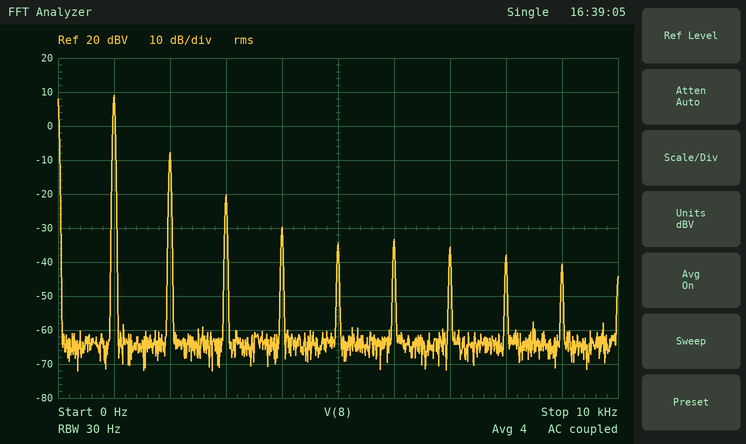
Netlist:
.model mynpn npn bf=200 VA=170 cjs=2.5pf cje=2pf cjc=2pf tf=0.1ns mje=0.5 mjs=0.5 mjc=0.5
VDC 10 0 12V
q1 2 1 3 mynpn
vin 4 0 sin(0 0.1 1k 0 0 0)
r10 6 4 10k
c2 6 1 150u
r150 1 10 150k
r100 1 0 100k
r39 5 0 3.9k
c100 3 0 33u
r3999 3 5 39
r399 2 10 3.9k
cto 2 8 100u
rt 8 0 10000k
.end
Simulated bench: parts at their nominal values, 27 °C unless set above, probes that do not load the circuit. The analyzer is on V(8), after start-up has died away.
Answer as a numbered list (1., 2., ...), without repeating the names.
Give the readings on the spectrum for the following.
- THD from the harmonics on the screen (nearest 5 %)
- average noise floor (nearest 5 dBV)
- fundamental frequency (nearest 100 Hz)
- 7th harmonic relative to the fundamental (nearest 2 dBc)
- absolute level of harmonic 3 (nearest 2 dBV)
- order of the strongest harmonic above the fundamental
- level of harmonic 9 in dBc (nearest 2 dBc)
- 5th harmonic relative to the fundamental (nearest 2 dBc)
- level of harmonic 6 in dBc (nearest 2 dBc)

1. 15 %
2. -65 dBV
3. 1.0 kHz
4. -44 dBc
5. -20 dBV
6. 2
7. -50 dBc
8. -44 dBc
9. -42 dBc
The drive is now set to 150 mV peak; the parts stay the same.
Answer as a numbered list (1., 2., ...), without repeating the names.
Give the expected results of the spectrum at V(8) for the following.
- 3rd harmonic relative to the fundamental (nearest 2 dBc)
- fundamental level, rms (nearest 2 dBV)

1. -16 dBc
2. 10 dBV
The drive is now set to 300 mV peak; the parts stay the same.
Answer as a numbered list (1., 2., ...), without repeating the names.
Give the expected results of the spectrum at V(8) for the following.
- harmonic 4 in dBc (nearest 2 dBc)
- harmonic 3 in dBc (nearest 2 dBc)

1. -20 dBc
2. -12 dBc
